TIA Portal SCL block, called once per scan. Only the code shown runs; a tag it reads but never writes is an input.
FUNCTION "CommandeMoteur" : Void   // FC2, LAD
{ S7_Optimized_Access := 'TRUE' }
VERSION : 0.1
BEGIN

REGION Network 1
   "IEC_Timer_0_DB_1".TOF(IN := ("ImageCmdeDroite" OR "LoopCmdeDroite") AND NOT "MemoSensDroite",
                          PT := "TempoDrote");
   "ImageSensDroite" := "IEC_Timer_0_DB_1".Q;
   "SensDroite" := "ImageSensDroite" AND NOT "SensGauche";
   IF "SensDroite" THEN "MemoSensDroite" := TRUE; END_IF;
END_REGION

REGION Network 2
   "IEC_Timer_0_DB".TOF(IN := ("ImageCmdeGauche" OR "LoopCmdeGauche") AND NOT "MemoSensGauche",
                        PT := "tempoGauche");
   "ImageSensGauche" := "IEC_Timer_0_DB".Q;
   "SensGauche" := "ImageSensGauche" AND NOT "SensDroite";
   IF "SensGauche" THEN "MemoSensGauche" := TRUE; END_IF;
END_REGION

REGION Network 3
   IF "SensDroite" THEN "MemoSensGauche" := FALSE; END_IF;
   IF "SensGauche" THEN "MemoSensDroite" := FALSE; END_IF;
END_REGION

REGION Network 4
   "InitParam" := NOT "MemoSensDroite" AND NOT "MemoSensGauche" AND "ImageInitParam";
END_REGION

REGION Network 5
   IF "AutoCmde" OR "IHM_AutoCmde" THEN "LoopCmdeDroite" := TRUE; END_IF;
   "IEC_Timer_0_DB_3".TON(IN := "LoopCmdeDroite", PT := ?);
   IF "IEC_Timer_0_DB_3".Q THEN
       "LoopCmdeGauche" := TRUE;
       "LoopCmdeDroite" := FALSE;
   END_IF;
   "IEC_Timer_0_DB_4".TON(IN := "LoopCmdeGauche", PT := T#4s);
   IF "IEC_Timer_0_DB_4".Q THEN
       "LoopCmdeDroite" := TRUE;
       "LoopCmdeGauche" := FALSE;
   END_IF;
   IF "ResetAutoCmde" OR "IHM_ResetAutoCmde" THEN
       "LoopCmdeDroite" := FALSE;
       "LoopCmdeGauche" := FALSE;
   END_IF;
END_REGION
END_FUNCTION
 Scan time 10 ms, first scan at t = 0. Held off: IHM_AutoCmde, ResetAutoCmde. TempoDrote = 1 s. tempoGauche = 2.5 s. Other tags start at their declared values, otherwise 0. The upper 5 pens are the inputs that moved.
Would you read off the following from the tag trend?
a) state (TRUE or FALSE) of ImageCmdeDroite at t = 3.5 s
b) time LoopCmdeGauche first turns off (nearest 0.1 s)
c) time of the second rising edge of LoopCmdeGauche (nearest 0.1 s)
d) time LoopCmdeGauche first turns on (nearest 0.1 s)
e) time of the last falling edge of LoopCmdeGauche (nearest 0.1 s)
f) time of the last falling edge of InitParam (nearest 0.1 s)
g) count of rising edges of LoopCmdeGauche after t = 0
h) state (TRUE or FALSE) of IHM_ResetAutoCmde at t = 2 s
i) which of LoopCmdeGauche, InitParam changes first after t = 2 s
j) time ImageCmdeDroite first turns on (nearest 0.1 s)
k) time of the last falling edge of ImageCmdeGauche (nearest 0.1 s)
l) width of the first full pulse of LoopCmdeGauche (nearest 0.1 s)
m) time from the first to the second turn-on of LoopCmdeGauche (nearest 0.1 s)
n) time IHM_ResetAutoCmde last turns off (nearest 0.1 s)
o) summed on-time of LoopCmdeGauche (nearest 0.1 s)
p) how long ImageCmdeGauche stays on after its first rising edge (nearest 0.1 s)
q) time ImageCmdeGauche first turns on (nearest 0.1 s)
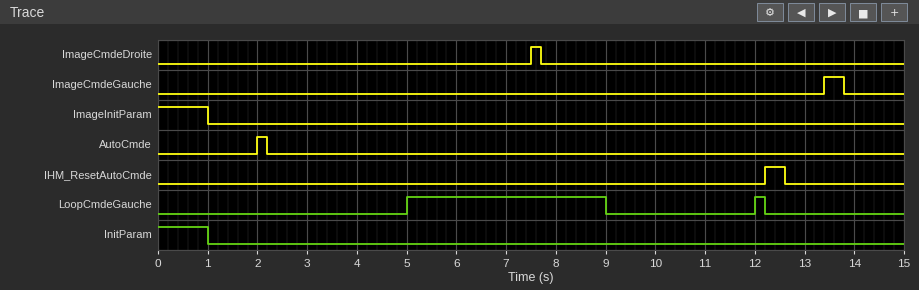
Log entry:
FALSE
9.0 s
12.0 s
5.0 s
12.2 s
1.0 s
2
FALSE
LoopCmdeGauche
7.5 s
13.8 s
4.0 s
7.0 s
12.6 s
4.2 s
0.4 s
13.4 s
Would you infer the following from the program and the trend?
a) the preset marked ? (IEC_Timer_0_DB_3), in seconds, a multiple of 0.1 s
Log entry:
3.0 s
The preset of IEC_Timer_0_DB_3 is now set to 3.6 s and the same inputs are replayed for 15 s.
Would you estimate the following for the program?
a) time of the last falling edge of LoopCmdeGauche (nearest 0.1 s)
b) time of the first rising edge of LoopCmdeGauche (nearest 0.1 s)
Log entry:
9.6 s
5.6 s
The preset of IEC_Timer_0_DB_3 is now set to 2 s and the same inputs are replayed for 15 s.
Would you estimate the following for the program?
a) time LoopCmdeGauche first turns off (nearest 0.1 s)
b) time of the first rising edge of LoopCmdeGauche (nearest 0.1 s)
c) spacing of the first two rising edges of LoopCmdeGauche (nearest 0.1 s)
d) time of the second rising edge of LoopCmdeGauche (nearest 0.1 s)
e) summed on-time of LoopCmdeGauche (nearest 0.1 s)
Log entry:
8.0 s
4.0 s
6.0 s
10.0 s
6.2 s
